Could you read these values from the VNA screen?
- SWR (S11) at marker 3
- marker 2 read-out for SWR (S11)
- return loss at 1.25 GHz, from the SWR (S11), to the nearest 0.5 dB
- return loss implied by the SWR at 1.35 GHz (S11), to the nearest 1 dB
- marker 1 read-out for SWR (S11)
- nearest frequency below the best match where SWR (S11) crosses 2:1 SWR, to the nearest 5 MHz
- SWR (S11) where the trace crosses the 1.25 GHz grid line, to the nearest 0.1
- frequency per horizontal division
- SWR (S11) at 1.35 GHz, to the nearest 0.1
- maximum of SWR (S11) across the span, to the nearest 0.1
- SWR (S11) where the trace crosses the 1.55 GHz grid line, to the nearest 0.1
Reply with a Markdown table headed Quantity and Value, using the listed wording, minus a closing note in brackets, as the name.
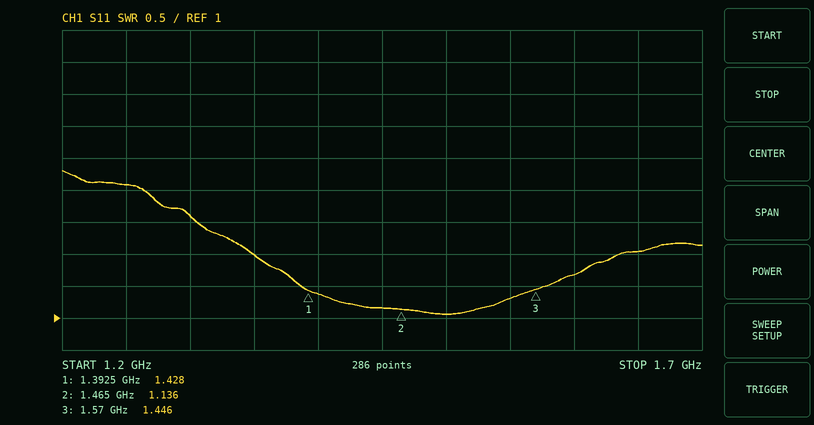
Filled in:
| Quantity | Value |
|---|---|
| SWR (S11) at marker 3 | 1.446 |
| marker 2 read-out for SWR | 1.136 |
| return loss at 1.25 GHz, from the SWR (S11), to the nearest 0.5 dB | 6.0 dB |
| return loss implied by the SWR at 1.35 GHz (S11), to the nearest 1 dB | 10 dB |
| marker 1 read-out for SWR | 1.428 |
| nearest frequency below the best match where SWR (S11) crosses 2:1 SWR, to the nearest 5 MHz | 1.350 GHz |
| SWR (S11) where the trace crosses the 1.25 GHz grid line, to the nearest 0.1 | 3.1 |
| frequency per horizontal division | 50 MHz |
| SWR (S11) at 1.35 GHz, to the nearest 0.1 | 2.0 |
| maximum of SWR (S11) across the span, to the nearest 0.1 | 3.3 |
| SWR (S11) where the trace crosses the 1.55 GHz grid line, to the nearest 0.1 | 1.3 |
